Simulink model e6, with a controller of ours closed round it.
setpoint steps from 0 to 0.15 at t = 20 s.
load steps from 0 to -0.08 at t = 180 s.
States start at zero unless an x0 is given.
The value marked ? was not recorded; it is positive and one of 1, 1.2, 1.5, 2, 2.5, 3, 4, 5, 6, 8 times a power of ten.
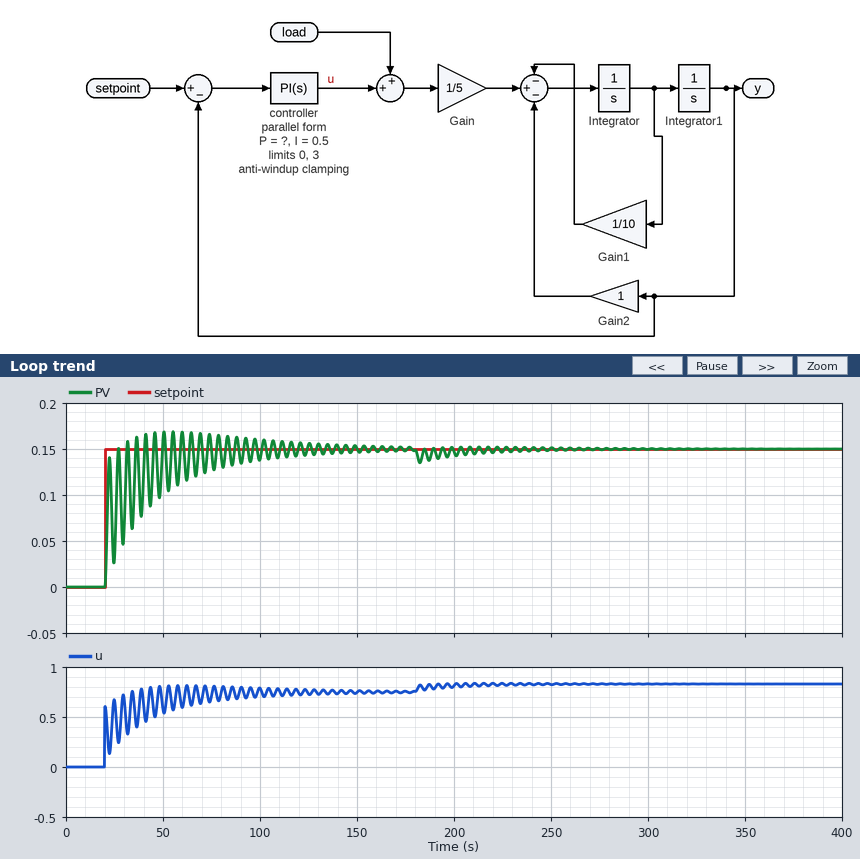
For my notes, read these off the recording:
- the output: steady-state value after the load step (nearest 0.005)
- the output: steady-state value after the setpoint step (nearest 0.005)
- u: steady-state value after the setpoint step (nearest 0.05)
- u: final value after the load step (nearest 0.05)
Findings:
0.150
0.150
0.75
0.85
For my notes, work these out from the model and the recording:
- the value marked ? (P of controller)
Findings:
4
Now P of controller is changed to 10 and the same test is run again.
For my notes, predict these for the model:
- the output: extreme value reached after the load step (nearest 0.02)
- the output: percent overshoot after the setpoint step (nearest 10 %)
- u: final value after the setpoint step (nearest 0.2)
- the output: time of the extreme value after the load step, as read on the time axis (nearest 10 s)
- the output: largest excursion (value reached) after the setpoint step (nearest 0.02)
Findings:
0.14
40 %
0.8
180 s
0.20
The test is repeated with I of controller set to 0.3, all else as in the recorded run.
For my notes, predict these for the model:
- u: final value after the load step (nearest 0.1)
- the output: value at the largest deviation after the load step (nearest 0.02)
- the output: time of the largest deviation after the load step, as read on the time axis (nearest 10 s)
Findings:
0.8
0.14
180 s
